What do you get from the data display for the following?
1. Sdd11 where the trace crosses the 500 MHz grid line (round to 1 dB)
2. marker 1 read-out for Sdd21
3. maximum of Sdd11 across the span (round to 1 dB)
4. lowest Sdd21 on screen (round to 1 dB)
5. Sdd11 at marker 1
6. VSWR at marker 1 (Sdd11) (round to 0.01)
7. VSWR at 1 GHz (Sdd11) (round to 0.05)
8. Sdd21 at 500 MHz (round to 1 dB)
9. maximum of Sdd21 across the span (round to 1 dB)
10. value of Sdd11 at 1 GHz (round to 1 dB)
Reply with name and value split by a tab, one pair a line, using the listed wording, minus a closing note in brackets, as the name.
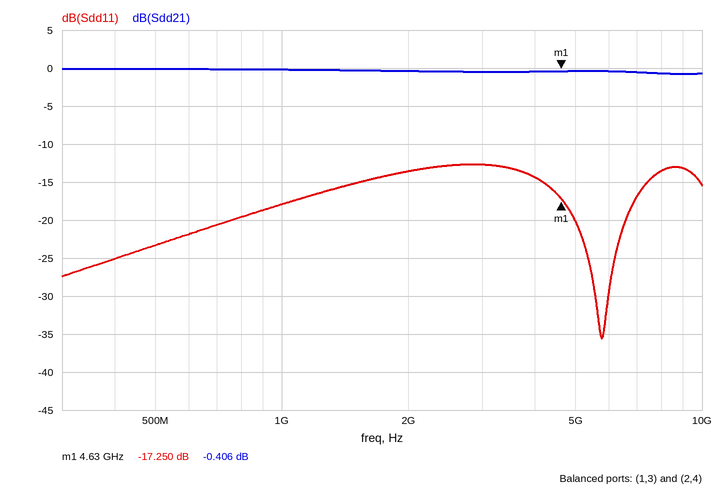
Sdd11 where the trace crosses the 500 MHz grid line	-23 dB
marker 1 read-out for Sdd21	-0.406 dB
maximum of Sdd11 across the span	-13 dB
lowest Sdd21 on screen	-1 dB
Sdd11 at marker 1	-17.250 dB
VSWR at marker 1 (Sdd11)	1.32
VSWR at 1 GHz (Sdd11)	1.30
Sdd21 at 500 MHz	0 dB
maximum of Sdd21 across the span	0 dB
value of Sdd11 at 1 GHz	-18 dB
